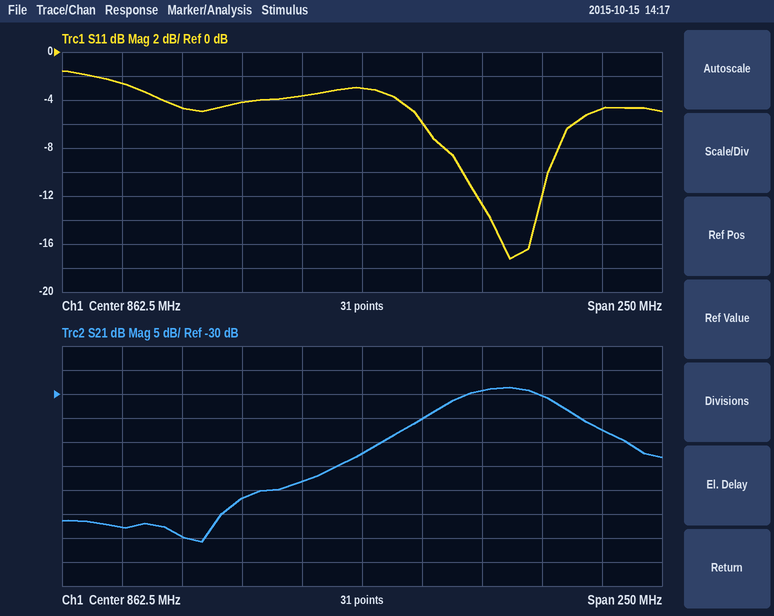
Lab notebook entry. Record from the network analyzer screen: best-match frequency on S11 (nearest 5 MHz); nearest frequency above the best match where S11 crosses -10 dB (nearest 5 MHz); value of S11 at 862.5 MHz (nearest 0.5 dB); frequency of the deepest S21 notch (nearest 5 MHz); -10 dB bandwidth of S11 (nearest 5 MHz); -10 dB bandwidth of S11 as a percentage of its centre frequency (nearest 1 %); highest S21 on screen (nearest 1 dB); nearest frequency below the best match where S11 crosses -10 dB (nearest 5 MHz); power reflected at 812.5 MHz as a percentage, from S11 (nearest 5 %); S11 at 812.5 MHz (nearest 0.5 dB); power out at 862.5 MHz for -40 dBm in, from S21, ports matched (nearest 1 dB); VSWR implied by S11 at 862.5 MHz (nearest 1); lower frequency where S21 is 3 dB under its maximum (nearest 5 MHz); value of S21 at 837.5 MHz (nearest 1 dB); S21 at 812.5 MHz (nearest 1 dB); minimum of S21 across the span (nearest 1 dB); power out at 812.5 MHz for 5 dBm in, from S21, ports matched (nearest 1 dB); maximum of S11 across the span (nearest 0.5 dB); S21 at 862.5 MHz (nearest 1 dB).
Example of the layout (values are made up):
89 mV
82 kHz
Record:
925 MHz
940 MHz
-3.0 dB
795 MHz
35 MHz
4 %
-29 dB
905 MHz
40 %
-4.0 dB
-82 dBm
6
900 MHz
-48 dB
-52 dB
-61 dB
-47 dBm
-1.5 dB
-42 dB
